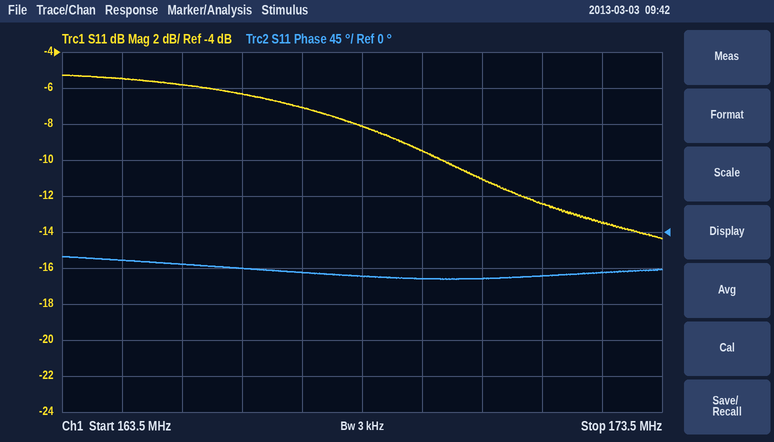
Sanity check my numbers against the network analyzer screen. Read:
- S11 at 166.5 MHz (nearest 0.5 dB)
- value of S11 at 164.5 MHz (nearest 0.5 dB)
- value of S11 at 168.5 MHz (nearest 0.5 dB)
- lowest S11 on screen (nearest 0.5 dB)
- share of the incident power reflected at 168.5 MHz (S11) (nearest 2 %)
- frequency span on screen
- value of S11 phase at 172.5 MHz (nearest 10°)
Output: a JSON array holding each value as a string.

["-6.5 dB", "-5.5 dB", "-8.0 dB", "-14.5 dB", "16 %", "10 MHz", "-50°"]
